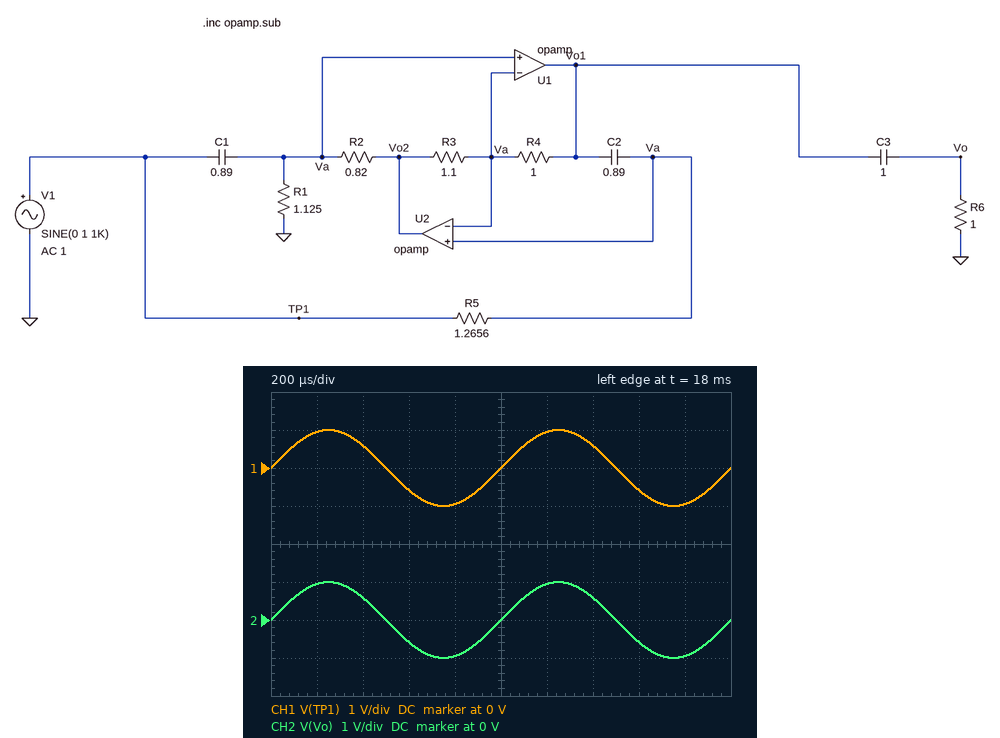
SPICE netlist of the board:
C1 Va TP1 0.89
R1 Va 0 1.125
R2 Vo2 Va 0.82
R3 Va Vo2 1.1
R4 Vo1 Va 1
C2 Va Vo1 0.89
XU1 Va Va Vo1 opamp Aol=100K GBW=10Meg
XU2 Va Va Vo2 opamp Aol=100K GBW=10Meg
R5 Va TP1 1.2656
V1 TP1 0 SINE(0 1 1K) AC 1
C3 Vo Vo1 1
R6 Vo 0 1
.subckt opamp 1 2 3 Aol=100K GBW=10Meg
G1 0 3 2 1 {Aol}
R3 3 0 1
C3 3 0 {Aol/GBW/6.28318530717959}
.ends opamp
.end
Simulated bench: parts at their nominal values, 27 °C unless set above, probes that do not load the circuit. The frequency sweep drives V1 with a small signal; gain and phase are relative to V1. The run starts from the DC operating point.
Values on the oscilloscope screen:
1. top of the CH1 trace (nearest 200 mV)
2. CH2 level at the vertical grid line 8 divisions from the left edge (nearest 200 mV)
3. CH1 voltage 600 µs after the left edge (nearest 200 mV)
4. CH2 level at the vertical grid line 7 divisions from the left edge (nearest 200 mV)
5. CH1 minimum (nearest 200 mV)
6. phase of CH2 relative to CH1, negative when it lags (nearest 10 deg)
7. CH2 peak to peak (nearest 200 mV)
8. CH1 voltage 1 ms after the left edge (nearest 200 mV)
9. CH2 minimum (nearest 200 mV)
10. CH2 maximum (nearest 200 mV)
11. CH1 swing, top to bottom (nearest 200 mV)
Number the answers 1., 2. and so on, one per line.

1. 1.0 V
2. -600 mV
3. -600 mV
4. 600 mV
5. -1.0 V
6. 0 deg
7. 2.0 V
8. 0 V
9. -1.0 V
10. 1.0 V
11. 2.0 V
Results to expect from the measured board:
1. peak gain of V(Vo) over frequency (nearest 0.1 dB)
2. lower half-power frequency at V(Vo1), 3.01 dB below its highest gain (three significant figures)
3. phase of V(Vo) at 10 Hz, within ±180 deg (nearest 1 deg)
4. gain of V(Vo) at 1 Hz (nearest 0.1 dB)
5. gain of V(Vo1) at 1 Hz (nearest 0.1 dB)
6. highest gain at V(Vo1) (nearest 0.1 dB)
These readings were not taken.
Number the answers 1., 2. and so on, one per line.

1. 0 dB
2. 1.10 Hz
3. 7 deg
4. -3.6 dB
5. -3.5 dB
6. 0 dB
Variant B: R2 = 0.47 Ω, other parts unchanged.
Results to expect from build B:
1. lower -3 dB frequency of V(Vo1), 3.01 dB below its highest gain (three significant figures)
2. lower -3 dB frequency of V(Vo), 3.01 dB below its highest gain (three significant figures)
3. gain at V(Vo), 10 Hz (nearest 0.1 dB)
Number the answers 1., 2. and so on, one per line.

1. 1.11 Hz
2. 1.14 Hz
3. -0.1 dB
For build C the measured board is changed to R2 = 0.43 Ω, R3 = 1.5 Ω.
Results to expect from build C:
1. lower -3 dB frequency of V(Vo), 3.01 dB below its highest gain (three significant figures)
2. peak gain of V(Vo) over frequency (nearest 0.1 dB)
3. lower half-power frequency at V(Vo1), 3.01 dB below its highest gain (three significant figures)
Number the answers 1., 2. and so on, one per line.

1. 1.14 Hz
2. 0 dB
3. 1.11 Hz
